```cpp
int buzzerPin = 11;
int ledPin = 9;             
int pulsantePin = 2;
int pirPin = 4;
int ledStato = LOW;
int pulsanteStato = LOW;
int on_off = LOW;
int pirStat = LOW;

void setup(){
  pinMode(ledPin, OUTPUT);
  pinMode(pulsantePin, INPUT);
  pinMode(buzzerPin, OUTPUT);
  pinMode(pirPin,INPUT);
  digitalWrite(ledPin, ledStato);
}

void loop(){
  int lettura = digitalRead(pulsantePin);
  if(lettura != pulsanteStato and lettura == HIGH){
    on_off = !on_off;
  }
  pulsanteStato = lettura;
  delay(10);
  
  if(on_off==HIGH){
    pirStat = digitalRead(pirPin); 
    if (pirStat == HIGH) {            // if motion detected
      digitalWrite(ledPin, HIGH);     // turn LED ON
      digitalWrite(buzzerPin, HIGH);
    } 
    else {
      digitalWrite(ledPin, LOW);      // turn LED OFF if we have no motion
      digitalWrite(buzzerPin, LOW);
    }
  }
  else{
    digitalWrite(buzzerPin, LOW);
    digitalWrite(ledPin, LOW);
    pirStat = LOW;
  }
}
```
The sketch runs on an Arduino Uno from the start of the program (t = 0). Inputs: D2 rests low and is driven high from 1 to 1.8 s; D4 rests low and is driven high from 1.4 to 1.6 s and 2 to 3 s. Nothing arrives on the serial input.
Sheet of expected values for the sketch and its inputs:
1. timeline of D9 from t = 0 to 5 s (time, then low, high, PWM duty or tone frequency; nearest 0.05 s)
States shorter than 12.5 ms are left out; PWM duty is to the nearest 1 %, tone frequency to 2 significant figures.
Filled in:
0 s low; 1.4 s high; 1.6 s low; 2 s high; 3 s low
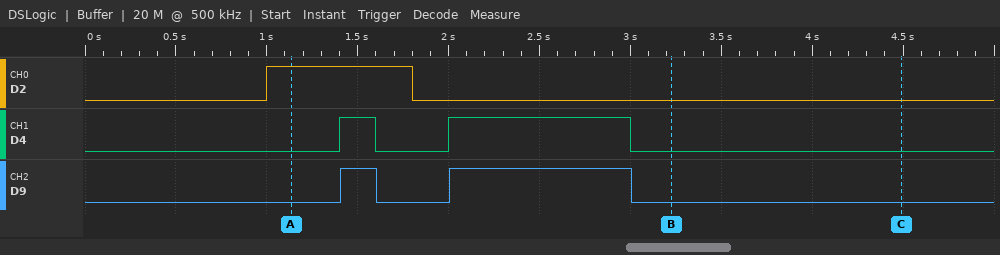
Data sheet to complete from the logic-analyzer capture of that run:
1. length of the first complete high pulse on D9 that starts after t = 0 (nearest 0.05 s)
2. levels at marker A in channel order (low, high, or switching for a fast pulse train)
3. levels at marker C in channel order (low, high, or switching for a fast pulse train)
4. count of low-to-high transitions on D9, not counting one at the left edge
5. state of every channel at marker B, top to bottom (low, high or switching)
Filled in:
0.20 s
D2 high, D4 low, D9 low
D2 low, D4 low, D9 low
2
D2 low, D4 low, D9 low
